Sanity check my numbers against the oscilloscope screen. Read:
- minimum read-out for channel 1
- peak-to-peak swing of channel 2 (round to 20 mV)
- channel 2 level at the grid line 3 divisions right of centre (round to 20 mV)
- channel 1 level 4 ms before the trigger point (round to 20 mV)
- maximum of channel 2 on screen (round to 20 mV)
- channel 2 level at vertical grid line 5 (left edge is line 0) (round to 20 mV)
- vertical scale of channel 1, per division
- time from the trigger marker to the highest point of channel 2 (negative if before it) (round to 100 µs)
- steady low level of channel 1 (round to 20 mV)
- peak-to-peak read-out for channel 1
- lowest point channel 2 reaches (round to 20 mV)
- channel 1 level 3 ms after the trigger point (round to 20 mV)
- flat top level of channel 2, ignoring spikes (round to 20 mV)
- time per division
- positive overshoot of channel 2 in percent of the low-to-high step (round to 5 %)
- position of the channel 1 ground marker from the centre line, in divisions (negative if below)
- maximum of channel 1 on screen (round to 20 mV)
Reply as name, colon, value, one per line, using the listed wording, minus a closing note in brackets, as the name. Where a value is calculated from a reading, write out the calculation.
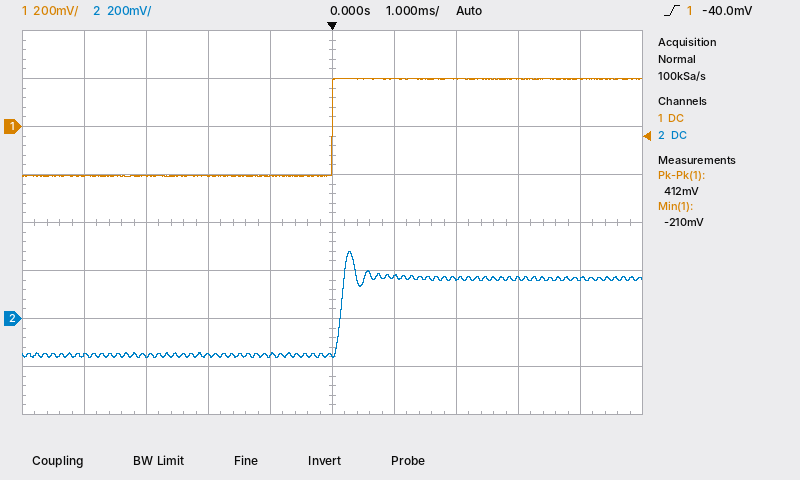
minimum read-out for channel 1: -210 mV
peak-to-peak swing of channel 2: 280 mV − (-160 mV) = 440 mV
channel 2 level at the grid line 3 divisions right of centre: 160 mV
channel 1 level 4 ms before the trigger point: -200 mV
maximum of channel 2 on screen: 280 mV
channel 2 level at vertical grid line 5 (left edge is line 0): -160 mV
vertical scale of channel 1, per division: 200 mV
time from the trigger marker to the highest point of channel 2 (negative if before it): +300 µs
steady low level of channel 1: -200 mV
peak-to-peak read-out for channel 1: 412 mV
lowest point channel 2 reaches: -160 mV
channel 1 level 3 ms after the trigger point: 200 mV
flat top level of channel 2, ignoring spikes: 160 mV
time per division: 1 ms
positive overshoot of channel 2 in percent of the low-to-high step: 35 %
position of the channel 1 ground marker from the centre line, in divisions: +2.0 div
maximum of channel 1 on screen: 200 mV
